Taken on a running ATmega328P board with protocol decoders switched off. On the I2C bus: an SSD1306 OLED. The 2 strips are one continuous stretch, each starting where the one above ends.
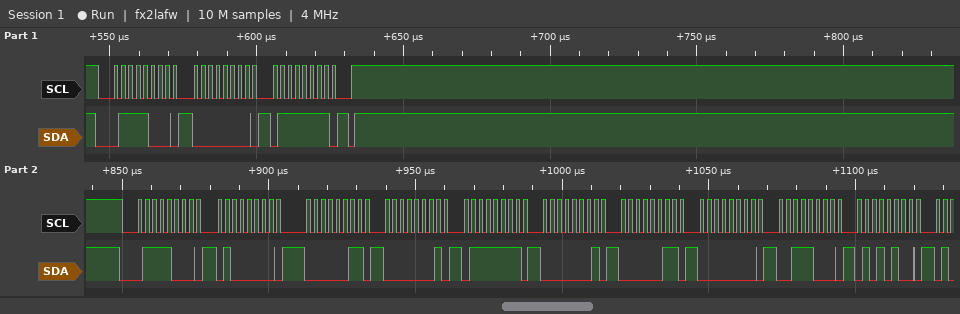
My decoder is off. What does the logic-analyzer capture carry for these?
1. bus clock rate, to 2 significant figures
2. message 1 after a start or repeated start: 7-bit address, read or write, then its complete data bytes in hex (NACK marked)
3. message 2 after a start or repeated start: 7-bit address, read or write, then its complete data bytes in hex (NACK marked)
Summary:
400 kHz
0x3C write: 00 7F
0x3C write: 40 03 01 7F 01 03 00 38 54
